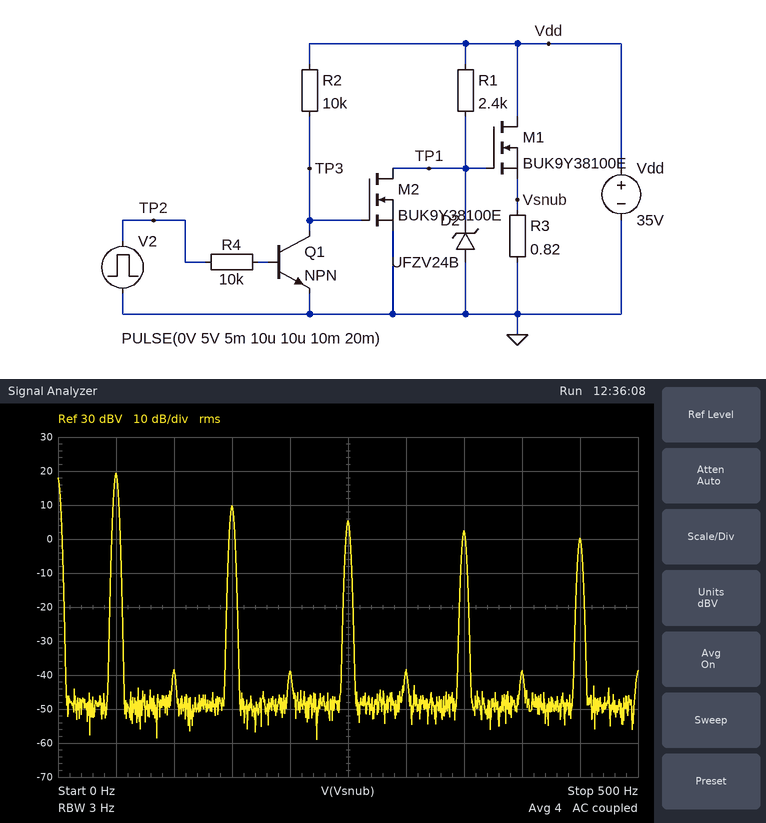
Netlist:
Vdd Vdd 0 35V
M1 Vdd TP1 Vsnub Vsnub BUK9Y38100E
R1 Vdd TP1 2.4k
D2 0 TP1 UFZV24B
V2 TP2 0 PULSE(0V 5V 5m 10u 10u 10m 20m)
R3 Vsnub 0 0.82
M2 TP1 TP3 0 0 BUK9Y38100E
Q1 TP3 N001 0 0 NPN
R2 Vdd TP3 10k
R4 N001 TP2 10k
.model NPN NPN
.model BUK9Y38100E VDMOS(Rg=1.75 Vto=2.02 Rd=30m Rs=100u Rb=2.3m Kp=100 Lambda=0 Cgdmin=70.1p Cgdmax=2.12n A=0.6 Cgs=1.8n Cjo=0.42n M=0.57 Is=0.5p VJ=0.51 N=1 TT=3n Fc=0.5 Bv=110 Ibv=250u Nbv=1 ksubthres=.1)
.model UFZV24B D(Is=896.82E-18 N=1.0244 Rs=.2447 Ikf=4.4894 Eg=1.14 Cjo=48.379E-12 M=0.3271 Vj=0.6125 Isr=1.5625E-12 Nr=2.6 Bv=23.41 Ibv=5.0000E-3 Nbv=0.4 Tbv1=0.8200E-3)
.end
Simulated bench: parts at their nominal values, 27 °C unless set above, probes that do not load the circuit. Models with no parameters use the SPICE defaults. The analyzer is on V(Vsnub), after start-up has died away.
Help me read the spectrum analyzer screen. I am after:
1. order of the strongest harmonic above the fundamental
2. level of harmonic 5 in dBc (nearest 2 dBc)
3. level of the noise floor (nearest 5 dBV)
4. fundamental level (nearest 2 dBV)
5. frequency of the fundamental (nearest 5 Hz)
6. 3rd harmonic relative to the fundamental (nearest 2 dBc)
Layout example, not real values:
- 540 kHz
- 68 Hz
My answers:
- 3
- -14 dBc
- -50 dBV
- 20 dBV
- 50 Hz
- -10 dBc
